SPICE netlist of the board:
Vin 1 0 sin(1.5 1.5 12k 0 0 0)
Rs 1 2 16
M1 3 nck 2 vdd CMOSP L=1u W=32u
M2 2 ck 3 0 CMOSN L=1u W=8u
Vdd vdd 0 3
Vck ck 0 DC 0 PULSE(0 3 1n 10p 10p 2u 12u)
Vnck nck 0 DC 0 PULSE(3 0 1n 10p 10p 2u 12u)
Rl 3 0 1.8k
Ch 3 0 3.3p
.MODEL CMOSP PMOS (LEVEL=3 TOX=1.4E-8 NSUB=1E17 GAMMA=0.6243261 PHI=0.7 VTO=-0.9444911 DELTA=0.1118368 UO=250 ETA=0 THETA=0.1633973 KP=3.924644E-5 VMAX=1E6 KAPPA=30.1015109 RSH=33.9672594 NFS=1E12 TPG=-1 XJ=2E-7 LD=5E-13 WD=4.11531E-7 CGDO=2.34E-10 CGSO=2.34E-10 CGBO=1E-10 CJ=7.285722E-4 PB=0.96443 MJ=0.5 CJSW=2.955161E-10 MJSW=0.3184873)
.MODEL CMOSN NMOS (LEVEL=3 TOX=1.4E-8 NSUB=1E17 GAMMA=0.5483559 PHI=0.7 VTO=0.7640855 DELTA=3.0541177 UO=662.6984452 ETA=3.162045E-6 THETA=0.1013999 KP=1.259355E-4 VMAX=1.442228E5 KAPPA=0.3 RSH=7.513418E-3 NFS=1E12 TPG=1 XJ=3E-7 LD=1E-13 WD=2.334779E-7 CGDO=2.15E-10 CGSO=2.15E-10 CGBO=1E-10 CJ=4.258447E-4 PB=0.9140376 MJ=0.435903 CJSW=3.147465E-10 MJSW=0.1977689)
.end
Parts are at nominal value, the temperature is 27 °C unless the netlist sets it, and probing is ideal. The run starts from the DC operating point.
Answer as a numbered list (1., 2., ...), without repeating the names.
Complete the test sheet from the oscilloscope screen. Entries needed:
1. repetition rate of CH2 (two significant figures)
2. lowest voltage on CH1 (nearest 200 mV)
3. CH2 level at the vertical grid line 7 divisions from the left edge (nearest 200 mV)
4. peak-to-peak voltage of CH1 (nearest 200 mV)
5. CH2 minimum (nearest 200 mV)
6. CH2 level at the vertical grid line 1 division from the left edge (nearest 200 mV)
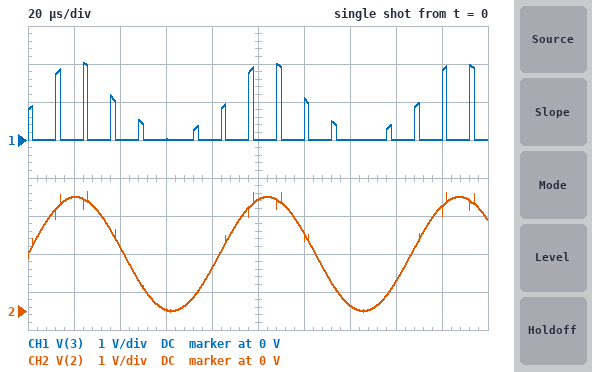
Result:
1. 12 kHz
2. 0 V
3. 200 mV
4. 2.0 V
5. 0 V
6. 3.0 V
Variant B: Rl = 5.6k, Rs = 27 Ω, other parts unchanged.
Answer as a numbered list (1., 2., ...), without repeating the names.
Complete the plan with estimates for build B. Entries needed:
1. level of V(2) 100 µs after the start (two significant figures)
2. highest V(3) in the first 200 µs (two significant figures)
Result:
1. 2.9 V
2. 2.6 V
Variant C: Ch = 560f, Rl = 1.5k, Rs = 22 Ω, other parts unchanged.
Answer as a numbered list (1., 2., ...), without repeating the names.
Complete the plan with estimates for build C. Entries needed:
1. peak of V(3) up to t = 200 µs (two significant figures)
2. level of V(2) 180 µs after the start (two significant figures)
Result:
1. 1.9 V
2. 2.8 V
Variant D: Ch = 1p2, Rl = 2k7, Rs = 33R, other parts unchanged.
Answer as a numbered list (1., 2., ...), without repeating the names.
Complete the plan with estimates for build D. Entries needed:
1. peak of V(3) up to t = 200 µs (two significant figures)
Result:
1. 2.3 V
